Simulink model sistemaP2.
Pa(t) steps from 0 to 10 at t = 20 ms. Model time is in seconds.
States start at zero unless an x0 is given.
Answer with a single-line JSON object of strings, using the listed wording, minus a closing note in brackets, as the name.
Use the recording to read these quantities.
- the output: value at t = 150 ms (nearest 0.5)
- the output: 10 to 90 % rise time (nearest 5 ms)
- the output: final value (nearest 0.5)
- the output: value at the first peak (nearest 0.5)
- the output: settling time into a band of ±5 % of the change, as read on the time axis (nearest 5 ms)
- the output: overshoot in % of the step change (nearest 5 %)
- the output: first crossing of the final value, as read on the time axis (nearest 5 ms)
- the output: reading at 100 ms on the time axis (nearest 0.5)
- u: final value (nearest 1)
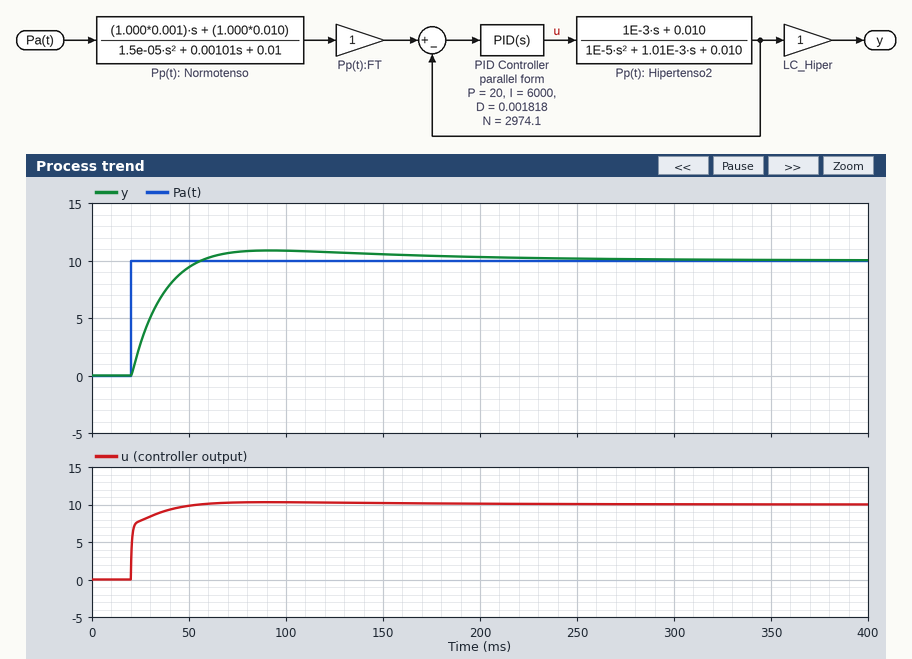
{"the output: value at t = 150 ms": "10.5", "the output: 10 to 90 % rise time": "25 ms", "the output: final value": "10.0", "the output: value at the first peak": "11.0", "the output: settling time into a band of ±5 % of the change, as read on the time axis": "155 ms", "the output: overshoot in % of the step change": "10 %", "the output: first crossing of the final value, as read on the time axis": "55 ms", "the output: reading at 100 ms on the time axis": "11.0", "u: final value": "10"}
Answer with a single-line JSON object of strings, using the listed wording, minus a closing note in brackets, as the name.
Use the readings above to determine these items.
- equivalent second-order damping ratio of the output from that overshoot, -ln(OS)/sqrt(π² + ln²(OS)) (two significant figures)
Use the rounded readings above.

{"equivalent second-order damping ratio of the output from that overshoot, -ln(OS)/sqrt(π² + ln²(OS))": "0.59"}
